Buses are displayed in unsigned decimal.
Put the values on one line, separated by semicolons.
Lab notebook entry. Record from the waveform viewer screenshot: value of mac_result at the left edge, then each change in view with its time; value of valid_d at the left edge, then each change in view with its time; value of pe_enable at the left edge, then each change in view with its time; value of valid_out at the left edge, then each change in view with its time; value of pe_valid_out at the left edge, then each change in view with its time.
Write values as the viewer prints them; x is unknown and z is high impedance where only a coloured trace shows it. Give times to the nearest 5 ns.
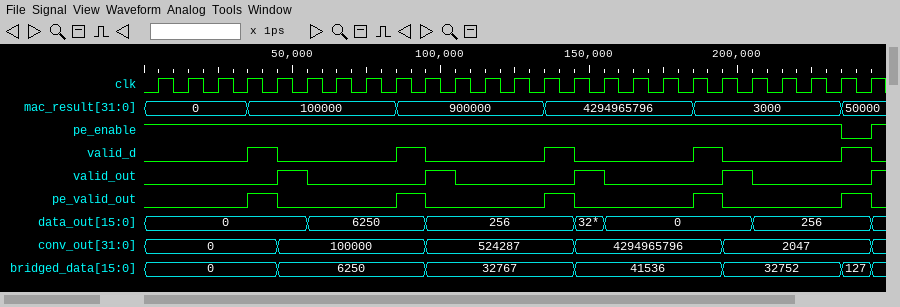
0, 100000 at 35 ns, 900000 at 85 ns, 4294965796 at 135 ns, 3000 at 185 ns, 50000 at 235 ns; 0, 1 at 35 ns, 0 at 45 ns, 1 at 85 ns, 0 at 95 ns, 1 at 135 ns, 0 at 145 ns, 1 at 185 ns, 0 at 195 ns, 1 at 235 ns, 0 at 245 ns; 1, 0 at 235 ns, 1 at 245 ns; 0, 1 at 45 ns, 0 at 55 ns, 1 at 95 ns, 0 at 105 ns, 1 at 145 ns, 0 at 155 ns, 1 at 195 ns, 0 at 205 ns, 1 at 245 ns; 0, 1 at 35 ns, 0 at 45 ns, 1 at 85 ns, 0 at 95 ns, 1 at 135 ns, 0 at 145 ns, 1 at 185 ns, 0 at 195 ns, 1 at 235 ns, 0 at 245 ns
